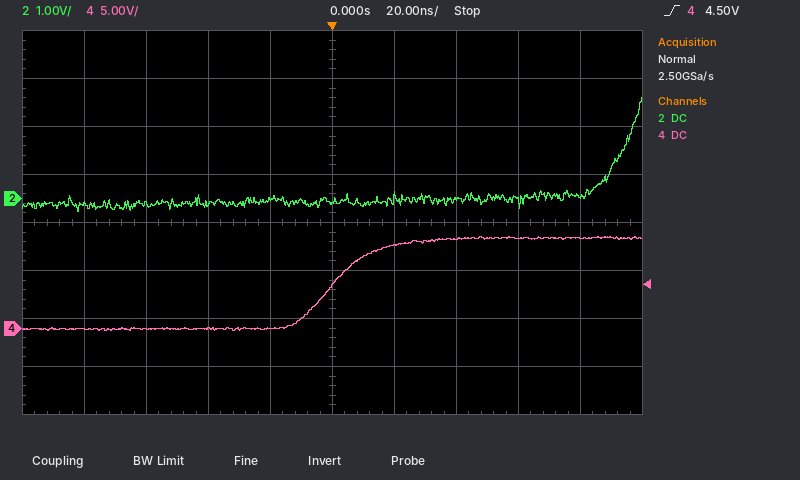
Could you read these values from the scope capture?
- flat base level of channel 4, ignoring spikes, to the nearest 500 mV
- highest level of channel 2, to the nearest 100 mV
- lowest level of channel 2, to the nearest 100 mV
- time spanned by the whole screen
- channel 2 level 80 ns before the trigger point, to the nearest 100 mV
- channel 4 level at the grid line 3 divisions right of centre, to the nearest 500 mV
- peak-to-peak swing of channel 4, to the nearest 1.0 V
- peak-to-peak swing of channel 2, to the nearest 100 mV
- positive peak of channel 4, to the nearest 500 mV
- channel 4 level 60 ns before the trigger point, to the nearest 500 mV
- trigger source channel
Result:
0.0 V
2.1 V
-300 mV
200 ns
-100 mV
9.5 V
10.0 V
2.4 V
9.5 V
0.0 V
channel 4
